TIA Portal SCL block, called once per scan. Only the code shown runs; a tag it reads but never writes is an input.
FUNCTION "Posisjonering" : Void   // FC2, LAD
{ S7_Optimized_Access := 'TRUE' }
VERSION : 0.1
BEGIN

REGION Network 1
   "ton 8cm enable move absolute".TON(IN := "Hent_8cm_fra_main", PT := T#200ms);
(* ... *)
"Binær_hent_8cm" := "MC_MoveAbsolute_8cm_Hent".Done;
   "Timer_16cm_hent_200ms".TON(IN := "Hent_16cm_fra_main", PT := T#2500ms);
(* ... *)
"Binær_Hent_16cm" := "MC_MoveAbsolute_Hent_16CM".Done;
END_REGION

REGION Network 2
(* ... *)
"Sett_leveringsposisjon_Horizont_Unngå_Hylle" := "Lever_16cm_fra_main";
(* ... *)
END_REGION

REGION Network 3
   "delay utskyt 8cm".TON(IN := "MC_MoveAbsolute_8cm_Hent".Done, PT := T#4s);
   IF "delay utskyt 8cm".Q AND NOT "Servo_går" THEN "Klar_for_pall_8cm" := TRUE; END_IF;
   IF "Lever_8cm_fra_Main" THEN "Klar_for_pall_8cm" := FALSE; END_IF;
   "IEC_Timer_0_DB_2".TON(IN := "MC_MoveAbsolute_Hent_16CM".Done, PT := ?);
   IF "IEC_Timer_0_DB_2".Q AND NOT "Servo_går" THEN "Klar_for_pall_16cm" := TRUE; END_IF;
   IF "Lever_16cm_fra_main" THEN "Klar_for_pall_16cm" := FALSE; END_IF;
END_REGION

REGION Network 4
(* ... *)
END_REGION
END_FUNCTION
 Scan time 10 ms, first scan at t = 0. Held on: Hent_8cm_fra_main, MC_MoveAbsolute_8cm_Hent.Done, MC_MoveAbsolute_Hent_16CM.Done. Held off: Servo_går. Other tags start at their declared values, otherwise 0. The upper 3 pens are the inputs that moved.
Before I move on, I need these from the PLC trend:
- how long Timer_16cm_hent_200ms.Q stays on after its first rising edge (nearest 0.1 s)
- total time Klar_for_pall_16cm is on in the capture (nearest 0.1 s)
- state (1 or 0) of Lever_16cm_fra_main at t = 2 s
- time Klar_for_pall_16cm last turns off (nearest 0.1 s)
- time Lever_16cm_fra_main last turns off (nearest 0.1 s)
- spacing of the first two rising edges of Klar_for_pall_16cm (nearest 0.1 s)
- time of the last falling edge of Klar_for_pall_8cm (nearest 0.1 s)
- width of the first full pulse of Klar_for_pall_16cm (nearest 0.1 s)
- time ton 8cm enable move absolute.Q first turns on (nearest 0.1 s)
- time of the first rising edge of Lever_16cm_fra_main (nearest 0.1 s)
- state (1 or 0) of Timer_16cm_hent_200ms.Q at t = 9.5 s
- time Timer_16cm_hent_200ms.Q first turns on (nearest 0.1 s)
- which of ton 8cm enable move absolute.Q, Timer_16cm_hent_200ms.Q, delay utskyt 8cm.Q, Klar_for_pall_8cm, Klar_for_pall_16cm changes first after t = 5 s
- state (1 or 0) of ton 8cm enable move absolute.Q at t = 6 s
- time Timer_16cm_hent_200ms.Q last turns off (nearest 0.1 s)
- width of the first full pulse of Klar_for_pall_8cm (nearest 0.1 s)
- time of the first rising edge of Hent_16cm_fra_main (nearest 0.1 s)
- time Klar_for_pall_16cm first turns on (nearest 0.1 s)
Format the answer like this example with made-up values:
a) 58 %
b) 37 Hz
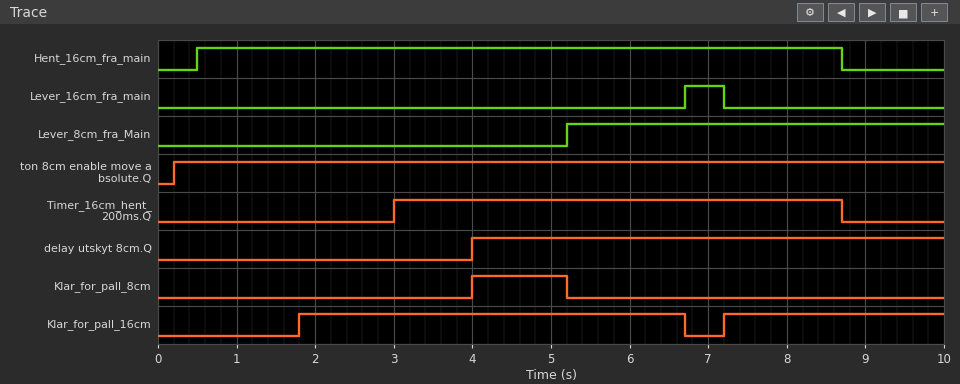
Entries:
a) 5.7 s
b) 7.7 s
c) 0
d) 6.7 s
e) 7.2 s
f) 5.4 s
g) 5.2 s
h) 4.9 s
i) 0.2 s
j) 6.7 s
k) 0
l) 3.0 s
m) Klar_for_pall_8cm
n) 1
o) 8.7 s
p) 1.2 s
q) 0.5 s
r) 1.8 s
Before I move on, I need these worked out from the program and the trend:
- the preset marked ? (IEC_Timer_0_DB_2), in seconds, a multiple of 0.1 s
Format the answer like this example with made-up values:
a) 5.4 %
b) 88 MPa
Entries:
a) 1.8 s
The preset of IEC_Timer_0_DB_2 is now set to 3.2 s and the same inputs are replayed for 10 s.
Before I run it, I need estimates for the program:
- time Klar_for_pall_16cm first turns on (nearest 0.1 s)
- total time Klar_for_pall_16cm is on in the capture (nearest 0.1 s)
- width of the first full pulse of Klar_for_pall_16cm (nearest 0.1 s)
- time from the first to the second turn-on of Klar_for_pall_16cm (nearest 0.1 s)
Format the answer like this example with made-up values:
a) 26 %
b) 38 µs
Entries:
a) 3.2 s
b) 6.3 s
c) 3.5 s
d) 4.0 s
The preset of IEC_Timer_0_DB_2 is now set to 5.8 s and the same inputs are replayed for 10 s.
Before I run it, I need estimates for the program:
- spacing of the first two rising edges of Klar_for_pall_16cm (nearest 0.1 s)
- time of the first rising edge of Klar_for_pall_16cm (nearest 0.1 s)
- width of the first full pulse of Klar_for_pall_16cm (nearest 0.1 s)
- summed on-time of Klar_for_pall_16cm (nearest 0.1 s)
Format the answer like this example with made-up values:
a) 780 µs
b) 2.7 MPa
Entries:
a) 1.4 s
b) 5.8 s
c) 0.9 s
d) 3.7 s
